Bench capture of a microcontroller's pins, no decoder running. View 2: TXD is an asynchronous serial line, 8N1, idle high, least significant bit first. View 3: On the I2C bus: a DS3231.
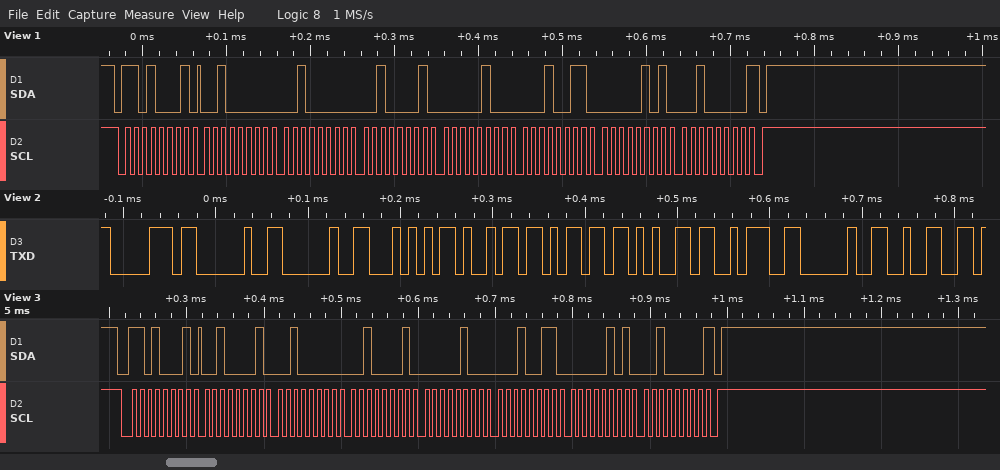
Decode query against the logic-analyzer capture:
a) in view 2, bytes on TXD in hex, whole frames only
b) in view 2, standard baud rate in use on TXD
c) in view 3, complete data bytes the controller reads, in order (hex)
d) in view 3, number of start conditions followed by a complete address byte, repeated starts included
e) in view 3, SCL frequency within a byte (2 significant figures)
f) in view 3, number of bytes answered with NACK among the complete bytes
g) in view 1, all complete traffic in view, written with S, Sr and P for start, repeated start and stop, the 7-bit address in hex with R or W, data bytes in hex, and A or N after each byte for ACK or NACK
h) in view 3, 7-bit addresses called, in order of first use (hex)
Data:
0x70 0x20 0x20 0x54 0x69 0x6D 0x65 0x3A 0x20 0x32
115200 baud
21 20 21 04 13 05 20
1
100 kHz
1
S 68R A 20 A 20 A 21 A 04 A 13 A 05 A 20 N P
0x68
